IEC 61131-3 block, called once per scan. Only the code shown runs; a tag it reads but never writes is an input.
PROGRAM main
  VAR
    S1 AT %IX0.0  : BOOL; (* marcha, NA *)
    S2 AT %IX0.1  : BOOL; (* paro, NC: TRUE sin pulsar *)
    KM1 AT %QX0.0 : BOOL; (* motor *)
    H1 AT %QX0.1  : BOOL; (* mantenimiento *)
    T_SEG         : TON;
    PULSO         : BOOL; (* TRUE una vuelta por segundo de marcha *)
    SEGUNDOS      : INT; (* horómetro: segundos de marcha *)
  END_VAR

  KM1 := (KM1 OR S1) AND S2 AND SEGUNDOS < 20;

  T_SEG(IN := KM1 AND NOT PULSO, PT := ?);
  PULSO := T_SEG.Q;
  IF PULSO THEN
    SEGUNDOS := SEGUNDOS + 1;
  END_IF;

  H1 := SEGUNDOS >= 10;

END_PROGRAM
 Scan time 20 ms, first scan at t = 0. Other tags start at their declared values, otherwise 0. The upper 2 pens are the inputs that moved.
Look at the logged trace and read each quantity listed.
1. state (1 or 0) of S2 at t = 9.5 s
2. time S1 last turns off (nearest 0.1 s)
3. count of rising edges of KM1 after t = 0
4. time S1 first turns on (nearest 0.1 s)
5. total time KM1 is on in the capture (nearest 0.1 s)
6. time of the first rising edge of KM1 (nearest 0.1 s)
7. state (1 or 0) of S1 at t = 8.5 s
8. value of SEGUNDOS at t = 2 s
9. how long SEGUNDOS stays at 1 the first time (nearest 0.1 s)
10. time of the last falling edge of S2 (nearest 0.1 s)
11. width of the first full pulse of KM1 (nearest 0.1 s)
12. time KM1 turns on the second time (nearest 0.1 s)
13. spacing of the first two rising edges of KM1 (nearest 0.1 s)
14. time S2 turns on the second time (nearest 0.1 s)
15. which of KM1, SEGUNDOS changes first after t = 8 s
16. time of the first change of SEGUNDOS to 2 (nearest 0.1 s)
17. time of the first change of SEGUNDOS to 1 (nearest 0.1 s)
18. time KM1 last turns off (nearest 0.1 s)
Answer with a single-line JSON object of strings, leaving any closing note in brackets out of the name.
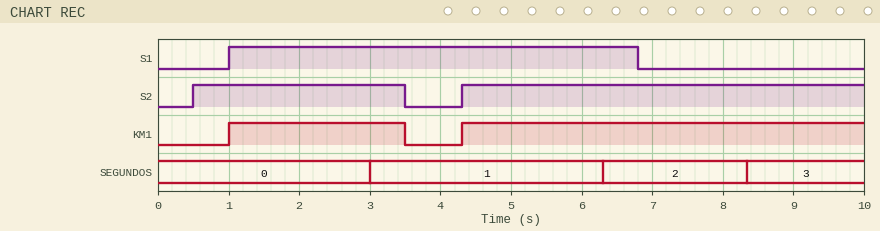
{"state (1 or 0) of S2 at t = 9.5 s": "1", "time S1 last turns off": "6.8 s", "count of rising edges of KM1 after t = 0": "2", "time S1 first turns on": "1.0 s", "total time KM1 is on in the capture": "8.2 s", "time of the first rising edge of KM1": "1.0 s", "state (1 or 0) of S1 at t = 8.5 s": "0", "value of SEGUNDOS at t = 2 s": "0", "how long SEGUNDOS stays at 1 the first time": "3.3 s", "time of the last falling edge of S2": "3.5 s", "width of the first full pulse of KM1": "2.5 s", "time KM1 turns on the second time": "4.3 s", "spacing of the first two rising edges of KM1": "3.3 s", "time S2 turns on the second time": "4.3 s", "which of KM1, SEGUNDOS changes first after t = 8 s": "SEGUNDOS", "time of the first change of SEGUNDOS to 2": "6.3 s", "time of the first change of SEGUNDOS to 1": "3.0 s", "time KM1 last turns off": "3.5 s"}
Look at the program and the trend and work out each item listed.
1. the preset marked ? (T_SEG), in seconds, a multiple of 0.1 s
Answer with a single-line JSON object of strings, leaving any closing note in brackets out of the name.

{"the preset marked ? (T_SEG), in seconds, a multiple of 0.1 s": "2.0 s"}
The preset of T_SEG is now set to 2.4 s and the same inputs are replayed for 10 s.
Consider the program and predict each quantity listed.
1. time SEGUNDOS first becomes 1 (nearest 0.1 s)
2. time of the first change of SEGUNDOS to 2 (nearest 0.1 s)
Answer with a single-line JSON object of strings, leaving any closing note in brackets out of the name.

{"time SEGUNDOS first becomes 1": "3.4 s", "time of the first change of SEGUNDOS to 2": "6.7 s"}
